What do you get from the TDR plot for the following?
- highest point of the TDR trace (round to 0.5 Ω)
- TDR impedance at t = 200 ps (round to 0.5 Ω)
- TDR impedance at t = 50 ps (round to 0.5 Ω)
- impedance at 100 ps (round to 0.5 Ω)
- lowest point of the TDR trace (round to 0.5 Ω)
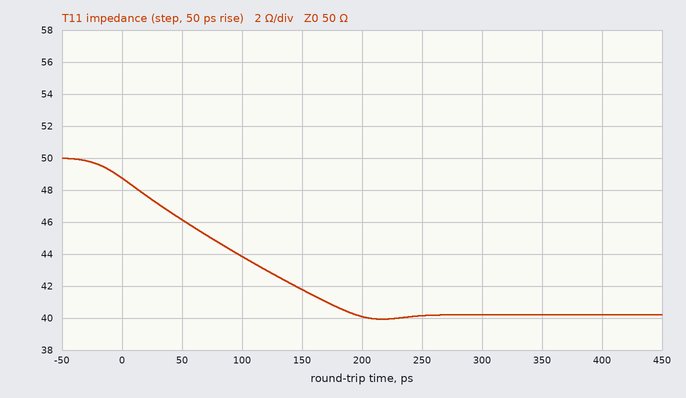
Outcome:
50.0 Ω
40.0 Ω
46.0 Ω
44.0 Ω
40.0 Ω
